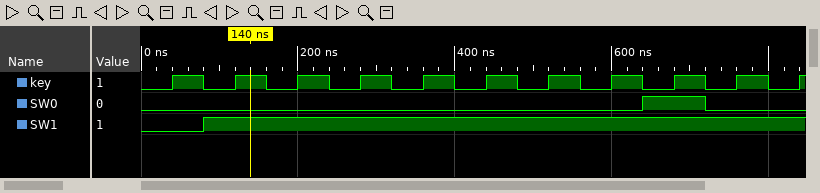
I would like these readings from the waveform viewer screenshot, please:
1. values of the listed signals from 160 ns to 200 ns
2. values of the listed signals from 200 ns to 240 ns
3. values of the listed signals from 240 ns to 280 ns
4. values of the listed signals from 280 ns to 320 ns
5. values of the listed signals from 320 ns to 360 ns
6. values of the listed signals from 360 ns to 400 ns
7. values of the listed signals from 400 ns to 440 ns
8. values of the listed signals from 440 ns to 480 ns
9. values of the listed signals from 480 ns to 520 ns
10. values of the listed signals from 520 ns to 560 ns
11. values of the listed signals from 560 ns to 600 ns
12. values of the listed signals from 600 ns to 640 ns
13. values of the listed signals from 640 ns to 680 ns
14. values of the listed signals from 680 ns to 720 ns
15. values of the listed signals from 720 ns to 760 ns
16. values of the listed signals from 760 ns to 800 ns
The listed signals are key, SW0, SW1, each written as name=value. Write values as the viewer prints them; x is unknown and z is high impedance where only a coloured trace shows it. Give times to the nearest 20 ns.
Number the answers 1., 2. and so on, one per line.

1. key=0, SW0=0, SW1=1
2. key=1, SW0=0, SW1=1
3. key=0, SW0=0, SW1=1
4. key=1, SW0=0, SW1=1
5. key=0, SW0=0, SW1=1
6. key=1, SW0=0, SW1=1
7. key=0, SW0=0, SW1=1
8. key=1, SW0=0, SW1=1
9. key=0, SW0=0, SW1=1
10. key=1, SW0=0, SW1=1
11. key=0, SW0=0, SW1=1
12. key=1, SW0=0, SW1=1
13. key=0, SW0=1, SW1=1
14. key=1, SW0=1, SW1=1
15. key=0, SW0=0, SW1=1
16. key=1, SW0=0, SW1=1
